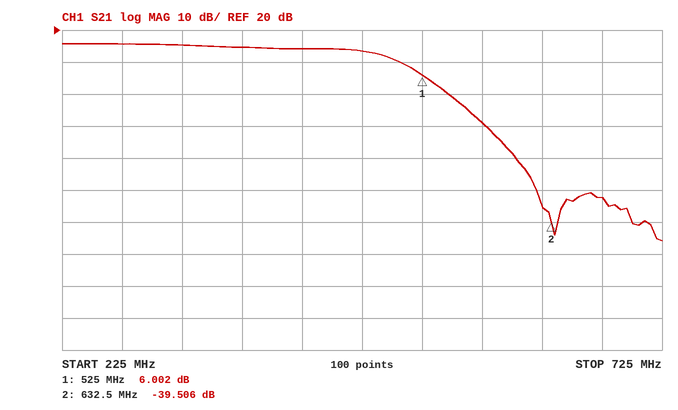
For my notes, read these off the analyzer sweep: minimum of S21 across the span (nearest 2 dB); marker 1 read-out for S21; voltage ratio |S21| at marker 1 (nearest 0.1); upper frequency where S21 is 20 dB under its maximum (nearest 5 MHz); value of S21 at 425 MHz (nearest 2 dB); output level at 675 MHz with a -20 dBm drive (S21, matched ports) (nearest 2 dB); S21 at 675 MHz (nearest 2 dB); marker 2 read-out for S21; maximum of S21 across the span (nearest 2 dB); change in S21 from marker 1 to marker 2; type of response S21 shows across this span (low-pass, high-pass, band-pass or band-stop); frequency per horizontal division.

-46 dB
6.002 dB
2.0
560 MHz
14 dB
-52 dBm
-32 dB
-39.506 dB
16 dB
-45.508 dB
low-pass
50 MHz
